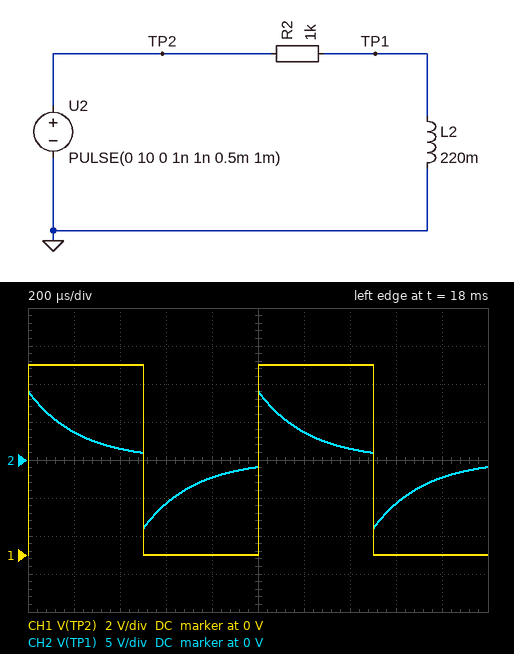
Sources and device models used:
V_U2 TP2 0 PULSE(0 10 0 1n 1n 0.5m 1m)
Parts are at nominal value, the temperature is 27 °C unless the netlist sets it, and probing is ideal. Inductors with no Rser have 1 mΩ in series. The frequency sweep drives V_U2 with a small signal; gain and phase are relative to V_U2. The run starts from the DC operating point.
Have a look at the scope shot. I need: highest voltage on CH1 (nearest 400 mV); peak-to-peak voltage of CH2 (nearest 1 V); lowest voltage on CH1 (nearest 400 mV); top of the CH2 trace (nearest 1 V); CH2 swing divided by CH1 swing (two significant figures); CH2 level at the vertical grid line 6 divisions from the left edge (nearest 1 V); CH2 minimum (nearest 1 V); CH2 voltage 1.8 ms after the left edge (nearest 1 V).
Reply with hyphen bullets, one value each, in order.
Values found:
- 10.0 V
- 18 V
- 0 V
- 9 V
- 1.8
- 4 V
- -9 V
- -2 V
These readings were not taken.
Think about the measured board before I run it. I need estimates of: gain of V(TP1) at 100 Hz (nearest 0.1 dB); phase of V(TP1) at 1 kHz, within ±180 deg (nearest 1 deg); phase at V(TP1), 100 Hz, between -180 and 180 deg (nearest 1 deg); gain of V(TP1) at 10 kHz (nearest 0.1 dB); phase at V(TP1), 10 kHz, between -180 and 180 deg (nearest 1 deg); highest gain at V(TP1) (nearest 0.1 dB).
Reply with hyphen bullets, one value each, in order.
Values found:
- -17.3 dB
- 36 deg
- 82 deg
- 0 dB
- 4 deg
- 0 dB
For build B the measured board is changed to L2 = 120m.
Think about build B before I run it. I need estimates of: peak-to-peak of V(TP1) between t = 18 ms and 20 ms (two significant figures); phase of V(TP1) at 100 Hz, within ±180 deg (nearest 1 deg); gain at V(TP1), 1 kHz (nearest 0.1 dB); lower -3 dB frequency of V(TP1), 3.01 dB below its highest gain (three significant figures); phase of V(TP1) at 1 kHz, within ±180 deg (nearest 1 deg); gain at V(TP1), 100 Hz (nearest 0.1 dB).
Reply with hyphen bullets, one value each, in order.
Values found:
- 20 V
- 86 deg
- -4.4 dB
- 1.33 kHz
- 53 deg
- -22.5 dB
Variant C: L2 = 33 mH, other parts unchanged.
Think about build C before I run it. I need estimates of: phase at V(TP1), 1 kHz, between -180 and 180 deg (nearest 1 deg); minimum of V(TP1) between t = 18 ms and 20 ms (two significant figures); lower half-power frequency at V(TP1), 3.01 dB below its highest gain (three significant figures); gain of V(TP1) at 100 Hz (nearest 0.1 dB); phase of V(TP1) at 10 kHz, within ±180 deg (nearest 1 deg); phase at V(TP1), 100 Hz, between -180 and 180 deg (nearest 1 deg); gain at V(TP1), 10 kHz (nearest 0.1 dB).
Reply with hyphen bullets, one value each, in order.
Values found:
- 78 deg
- -10 V
- 4.82 kHz
- -33.7 dB
- 26 deg
- 89 deg
- -0.9 dB
